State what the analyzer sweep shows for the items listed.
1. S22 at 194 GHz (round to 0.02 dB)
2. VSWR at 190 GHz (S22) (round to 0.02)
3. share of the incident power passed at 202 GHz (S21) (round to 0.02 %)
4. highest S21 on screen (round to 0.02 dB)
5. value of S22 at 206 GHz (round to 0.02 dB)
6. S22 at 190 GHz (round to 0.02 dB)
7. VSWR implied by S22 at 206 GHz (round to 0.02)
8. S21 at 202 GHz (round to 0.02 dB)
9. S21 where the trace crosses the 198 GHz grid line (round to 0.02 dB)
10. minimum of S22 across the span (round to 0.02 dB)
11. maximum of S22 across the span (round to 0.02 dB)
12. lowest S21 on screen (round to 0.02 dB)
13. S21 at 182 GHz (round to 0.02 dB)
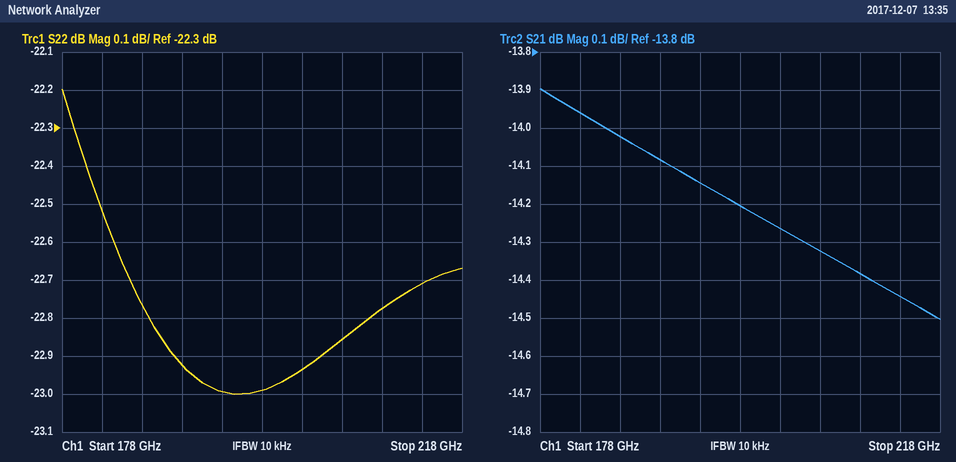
-23.00 dB
1.16
3.74 %
-13.90 dB
-22.86 dB
-22.92 dB
1.16
-14.26 dB
-14.20 dB
-23.00 dB
-22.20 dB
-14.50 dB
-13.96 dB
